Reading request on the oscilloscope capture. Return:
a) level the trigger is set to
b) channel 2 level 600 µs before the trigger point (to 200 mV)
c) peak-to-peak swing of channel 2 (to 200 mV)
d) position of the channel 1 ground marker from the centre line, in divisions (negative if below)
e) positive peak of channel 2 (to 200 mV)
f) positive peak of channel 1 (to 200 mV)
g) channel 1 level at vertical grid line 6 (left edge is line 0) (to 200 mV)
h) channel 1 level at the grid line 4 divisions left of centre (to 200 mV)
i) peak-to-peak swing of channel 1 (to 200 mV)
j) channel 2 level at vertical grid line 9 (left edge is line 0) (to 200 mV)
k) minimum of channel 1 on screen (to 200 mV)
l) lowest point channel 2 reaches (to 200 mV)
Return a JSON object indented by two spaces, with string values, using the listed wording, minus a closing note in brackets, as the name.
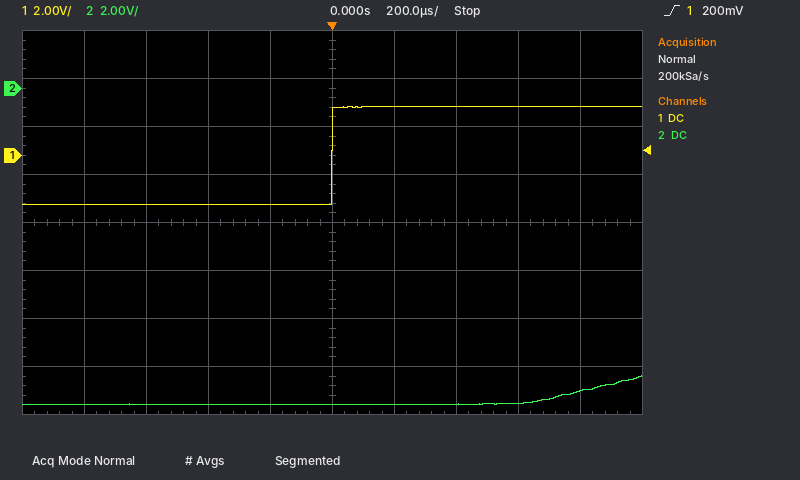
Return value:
{
  "level the trigger is set to": "200 mV",
  "channel 2 level 600 µs before the trigger point": "-13.2 V",
  "peak-to-peak swing of channel 2": "1.2 V",
  "position of the channel 1 ground marker from the centre line, in divisions": "+1.4 div",
  "positive peak of channel 2": "-12.0 V",
  "positive peak of channel 1": "2.0 V",
  "channel 1 level at vertical grid line 6 (left edge is line 0)": "2.0 V",
  "channel 1 level at the grid line 4 divisions left of centre": "-2.0 V",
  "peak-to-peak swing of channel 1": "4.0 V",
  "channel 2 level at vertical grid line 9 (left edge is line 0)": "-12.6 V",
  "minimum of channel 1 on screen": "-2.0 V",
  "lowest point channel 2 reaches": "-13.2 V"
}
